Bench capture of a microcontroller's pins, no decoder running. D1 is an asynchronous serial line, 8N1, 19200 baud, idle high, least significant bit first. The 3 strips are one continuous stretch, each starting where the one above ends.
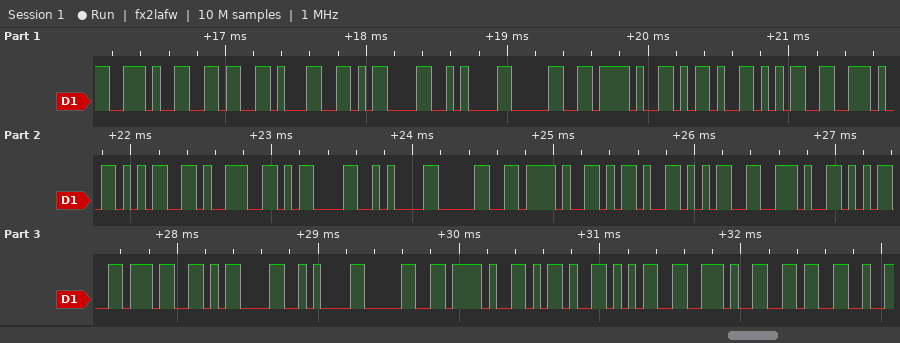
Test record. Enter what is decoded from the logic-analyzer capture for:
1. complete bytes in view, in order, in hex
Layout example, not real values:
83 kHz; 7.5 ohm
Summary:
0x2E 0x36 0x31 0x0D 0x0A 0x30 0x2F 0x2D 0x35 0x2E 0x35 0x39 0x0D 0x0A 0x30 0x2F 0x2D 0x35 0x2E 0x35 0x37 0x0D 0x0A 0x30 0x2F 0x2D 0x35 0x2E 0x36
